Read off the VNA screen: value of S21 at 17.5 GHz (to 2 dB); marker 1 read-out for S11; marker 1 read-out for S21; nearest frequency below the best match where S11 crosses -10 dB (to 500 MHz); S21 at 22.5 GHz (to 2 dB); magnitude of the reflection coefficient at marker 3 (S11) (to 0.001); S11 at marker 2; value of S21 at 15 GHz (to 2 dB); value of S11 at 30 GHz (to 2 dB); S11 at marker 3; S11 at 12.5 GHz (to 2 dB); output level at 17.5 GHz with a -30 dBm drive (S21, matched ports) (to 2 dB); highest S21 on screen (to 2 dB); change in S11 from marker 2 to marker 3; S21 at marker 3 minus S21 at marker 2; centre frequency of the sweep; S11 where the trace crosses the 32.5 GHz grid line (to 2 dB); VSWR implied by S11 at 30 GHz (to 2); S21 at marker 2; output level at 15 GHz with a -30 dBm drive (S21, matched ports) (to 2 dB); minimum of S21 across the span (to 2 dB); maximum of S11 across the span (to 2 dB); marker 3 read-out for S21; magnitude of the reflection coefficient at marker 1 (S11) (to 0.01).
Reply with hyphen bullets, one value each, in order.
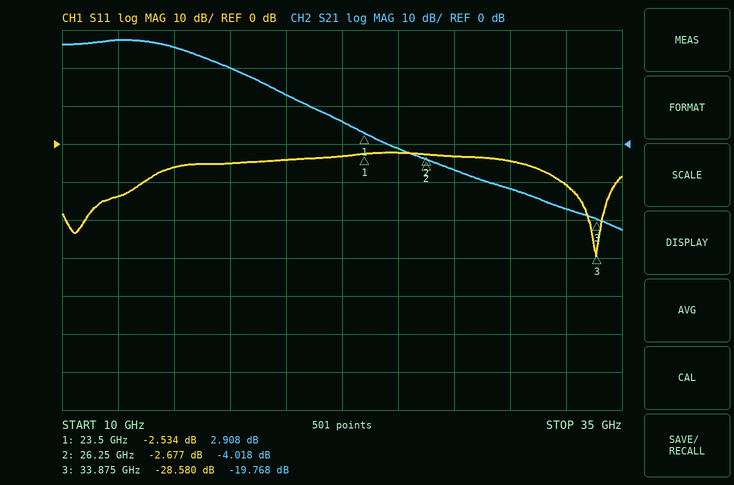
- 20 dB
- -2.534 dB
- 2.908 dB
- 32.5 GHz
- 6 dB
- 0.037
- -2.677 dB
- 26 dB
- -4 dB
- -28.580 dB
- -14 dB
- -10 dBm
- 28 dB
- -25.903 dB
- -15.750 dB
- 22.5 GHz
- -10 dB
- 4
- -4.018 dB
- -4 dBm
- -22 dB
- -2 dB
- -19.768 dB
- 0.75
